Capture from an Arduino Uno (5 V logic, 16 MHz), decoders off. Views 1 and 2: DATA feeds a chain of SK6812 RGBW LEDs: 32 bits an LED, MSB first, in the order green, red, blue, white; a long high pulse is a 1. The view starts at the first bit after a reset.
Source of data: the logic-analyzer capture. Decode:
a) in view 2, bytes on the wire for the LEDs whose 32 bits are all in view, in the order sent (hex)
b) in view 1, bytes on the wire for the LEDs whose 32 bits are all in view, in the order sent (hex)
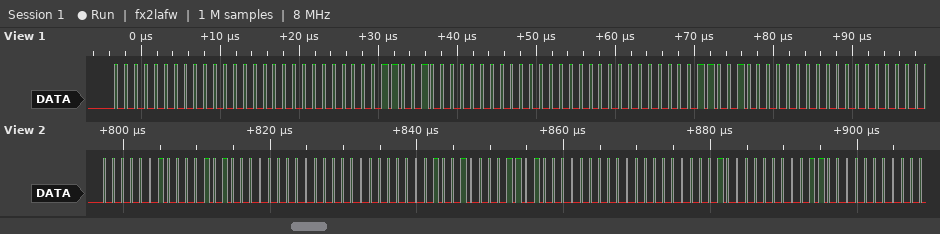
02 14 00 00 09 0D 00 00
00 00 00 19 00 00 00 19
